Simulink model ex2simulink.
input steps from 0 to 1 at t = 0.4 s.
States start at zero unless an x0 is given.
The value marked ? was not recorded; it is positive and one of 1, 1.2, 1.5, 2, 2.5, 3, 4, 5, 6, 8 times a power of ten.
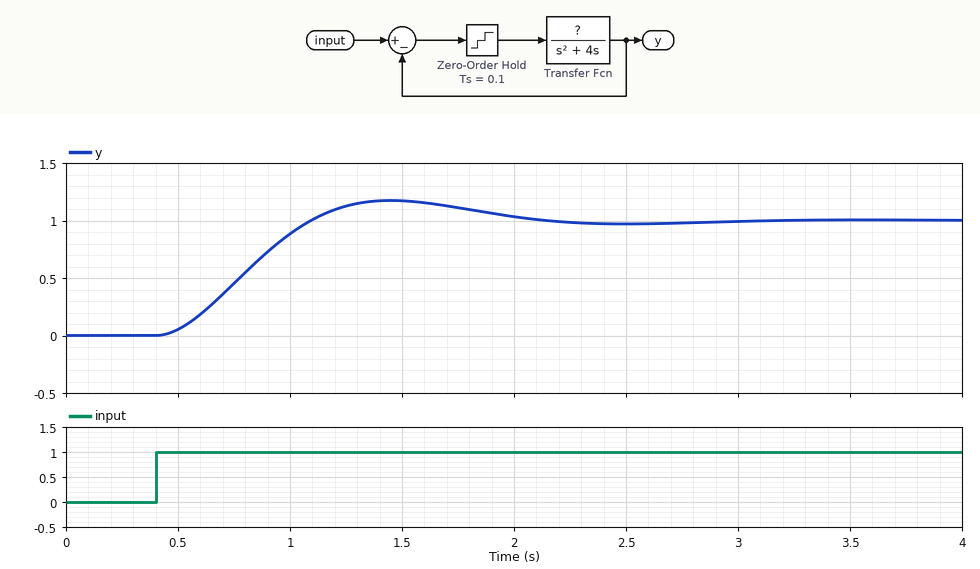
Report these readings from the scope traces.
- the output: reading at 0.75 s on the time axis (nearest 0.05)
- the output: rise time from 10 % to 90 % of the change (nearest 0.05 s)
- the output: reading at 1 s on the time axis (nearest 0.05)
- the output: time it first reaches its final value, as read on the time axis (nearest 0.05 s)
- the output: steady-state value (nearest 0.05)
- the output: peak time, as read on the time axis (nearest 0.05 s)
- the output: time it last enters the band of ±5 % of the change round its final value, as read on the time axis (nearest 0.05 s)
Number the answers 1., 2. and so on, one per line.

1. 0.45
2. 0.45 s
3. 0.90
4. 1.10 s
5. 1.00
6. 1.45 s
7. 1.95 s
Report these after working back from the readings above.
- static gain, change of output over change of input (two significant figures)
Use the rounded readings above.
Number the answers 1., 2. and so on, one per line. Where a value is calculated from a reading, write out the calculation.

1. (1 - 0) / (1 - 0) = 1.0
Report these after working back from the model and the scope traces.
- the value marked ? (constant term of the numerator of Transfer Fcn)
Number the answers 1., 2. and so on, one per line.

1. 12
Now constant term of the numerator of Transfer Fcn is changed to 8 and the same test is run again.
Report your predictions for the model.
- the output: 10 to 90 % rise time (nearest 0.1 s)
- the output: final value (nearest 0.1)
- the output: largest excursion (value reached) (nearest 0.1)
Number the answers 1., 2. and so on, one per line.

1. 0.7 s
2. 1.0
3. 1.1
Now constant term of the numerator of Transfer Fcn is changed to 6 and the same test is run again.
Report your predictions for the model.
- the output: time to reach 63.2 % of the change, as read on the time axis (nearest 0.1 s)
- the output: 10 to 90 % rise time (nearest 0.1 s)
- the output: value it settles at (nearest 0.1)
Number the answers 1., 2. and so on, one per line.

1. 1.1 s
2. 0.9 s
3. 1.0
